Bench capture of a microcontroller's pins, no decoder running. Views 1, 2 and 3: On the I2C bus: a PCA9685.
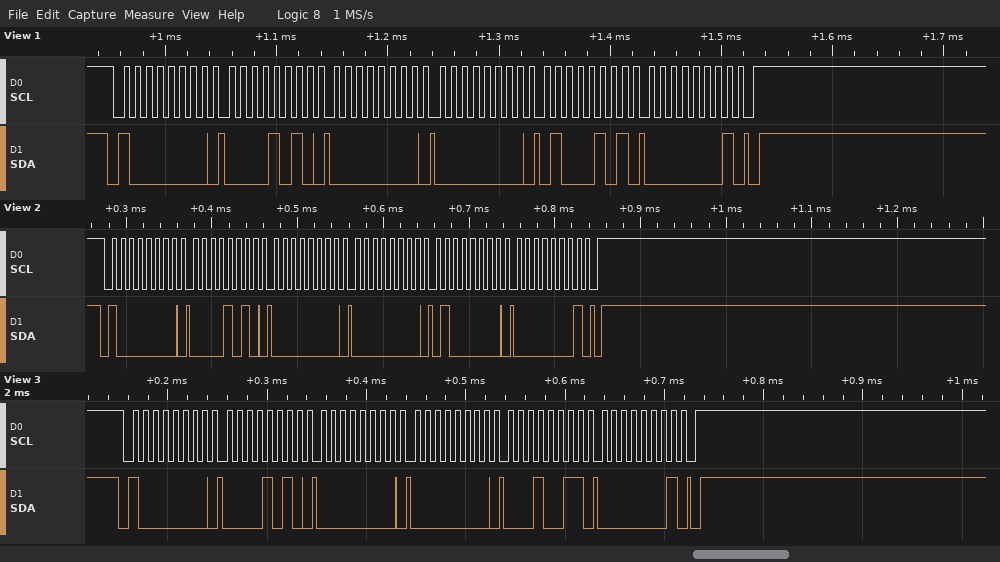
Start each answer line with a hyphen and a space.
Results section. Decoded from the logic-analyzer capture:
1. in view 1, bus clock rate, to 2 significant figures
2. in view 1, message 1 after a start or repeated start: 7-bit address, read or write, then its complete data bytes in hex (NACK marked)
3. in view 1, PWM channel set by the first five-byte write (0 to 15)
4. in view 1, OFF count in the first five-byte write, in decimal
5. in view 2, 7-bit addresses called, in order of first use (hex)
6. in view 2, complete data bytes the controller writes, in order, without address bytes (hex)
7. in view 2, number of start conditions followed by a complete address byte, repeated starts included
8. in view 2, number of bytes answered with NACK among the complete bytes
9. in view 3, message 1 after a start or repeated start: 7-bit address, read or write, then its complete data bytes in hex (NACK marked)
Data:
- 100 kHz
- 0x40 write: 0A 00 00 45 01
- 1
- 325
- 0x40
- 0A 00 00 40 01
- 1
- 0
- 0x40 write: 0A 00 00 13 01
